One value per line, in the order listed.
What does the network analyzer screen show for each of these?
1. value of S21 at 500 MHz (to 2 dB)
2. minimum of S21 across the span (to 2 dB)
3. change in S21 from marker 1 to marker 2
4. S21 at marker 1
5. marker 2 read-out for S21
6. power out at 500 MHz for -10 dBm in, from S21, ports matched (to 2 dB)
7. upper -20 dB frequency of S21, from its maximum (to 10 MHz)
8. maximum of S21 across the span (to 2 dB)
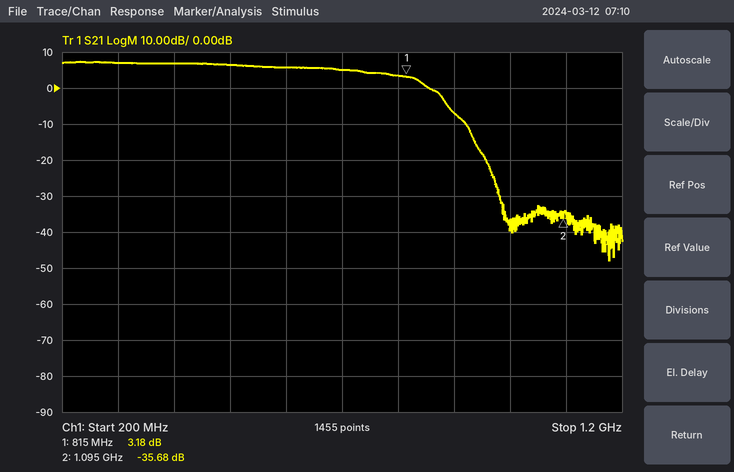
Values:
6 dB
-48 dB
-38.86 dB
3.18 dB
-35.68 dB
-4 dBm
930 MHz
8 dB
